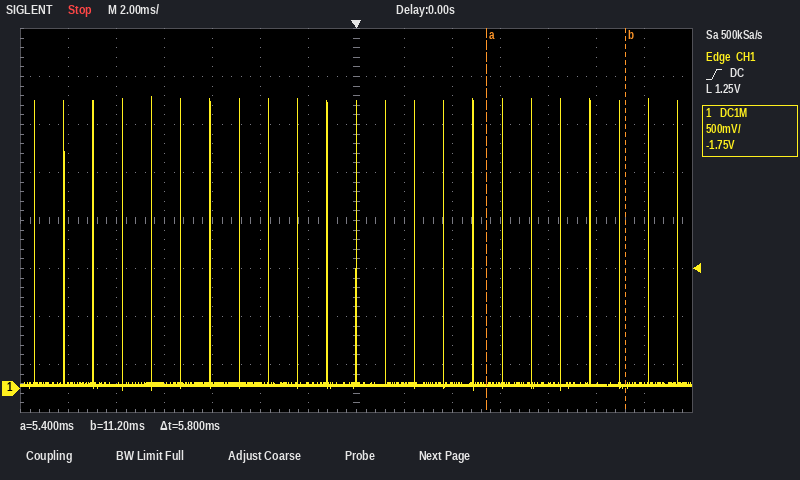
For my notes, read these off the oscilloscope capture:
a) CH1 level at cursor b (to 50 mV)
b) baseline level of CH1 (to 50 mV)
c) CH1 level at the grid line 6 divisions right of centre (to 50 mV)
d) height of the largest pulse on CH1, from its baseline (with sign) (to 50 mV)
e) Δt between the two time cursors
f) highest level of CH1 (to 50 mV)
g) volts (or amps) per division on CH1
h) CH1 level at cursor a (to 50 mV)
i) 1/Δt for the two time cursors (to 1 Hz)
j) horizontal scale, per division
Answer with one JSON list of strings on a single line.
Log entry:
["50 mV", "50 mV", "50 mV", "+3.00 V", "5.8 ms", "3.05 V", "500 mV", "50 mV", "172 Hz", "2 ms"]
